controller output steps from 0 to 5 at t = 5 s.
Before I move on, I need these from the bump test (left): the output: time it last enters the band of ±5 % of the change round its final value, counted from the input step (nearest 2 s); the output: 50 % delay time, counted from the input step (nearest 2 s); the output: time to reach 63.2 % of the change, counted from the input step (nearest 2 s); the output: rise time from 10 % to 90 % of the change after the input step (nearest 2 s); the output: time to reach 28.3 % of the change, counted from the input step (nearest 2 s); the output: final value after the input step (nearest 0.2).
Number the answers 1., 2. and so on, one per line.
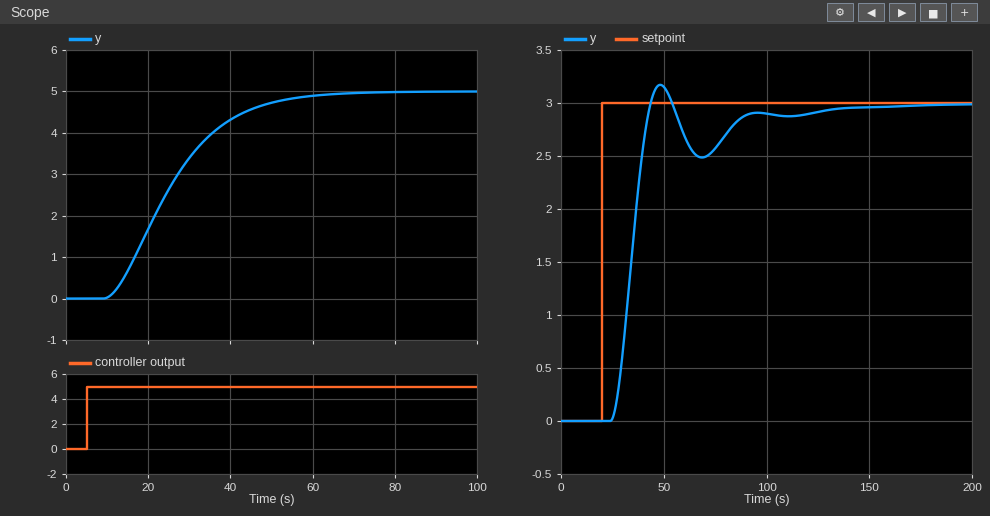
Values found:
1. 46 s
2. 20 s
3. 24 s
4. 30 s
5. 14 s
6. 5.0
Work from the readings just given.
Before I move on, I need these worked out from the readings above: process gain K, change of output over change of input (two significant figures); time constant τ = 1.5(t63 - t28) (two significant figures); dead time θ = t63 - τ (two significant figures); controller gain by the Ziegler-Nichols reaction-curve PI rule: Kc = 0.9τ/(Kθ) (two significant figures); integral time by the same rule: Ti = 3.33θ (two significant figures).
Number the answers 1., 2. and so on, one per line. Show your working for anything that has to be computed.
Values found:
1. (5 - 0) / 5 = 1.0
2. 1.5 × (24 - 14) = 15 s
3. 24 - 15 = 9.0 s
4. 0.9 × 15 / (1 × 9) = 1.5
5. 3.33 × 9 = 30 s
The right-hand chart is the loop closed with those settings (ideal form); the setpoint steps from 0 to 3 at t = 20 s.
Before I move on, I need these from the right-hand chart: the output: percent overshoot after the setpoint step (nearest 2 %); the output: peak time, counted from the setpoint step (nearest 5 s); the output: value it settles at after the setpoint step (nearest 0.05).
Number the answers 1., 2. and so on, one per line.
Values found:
1. 6 %
2. 30 s
3. 3.00
